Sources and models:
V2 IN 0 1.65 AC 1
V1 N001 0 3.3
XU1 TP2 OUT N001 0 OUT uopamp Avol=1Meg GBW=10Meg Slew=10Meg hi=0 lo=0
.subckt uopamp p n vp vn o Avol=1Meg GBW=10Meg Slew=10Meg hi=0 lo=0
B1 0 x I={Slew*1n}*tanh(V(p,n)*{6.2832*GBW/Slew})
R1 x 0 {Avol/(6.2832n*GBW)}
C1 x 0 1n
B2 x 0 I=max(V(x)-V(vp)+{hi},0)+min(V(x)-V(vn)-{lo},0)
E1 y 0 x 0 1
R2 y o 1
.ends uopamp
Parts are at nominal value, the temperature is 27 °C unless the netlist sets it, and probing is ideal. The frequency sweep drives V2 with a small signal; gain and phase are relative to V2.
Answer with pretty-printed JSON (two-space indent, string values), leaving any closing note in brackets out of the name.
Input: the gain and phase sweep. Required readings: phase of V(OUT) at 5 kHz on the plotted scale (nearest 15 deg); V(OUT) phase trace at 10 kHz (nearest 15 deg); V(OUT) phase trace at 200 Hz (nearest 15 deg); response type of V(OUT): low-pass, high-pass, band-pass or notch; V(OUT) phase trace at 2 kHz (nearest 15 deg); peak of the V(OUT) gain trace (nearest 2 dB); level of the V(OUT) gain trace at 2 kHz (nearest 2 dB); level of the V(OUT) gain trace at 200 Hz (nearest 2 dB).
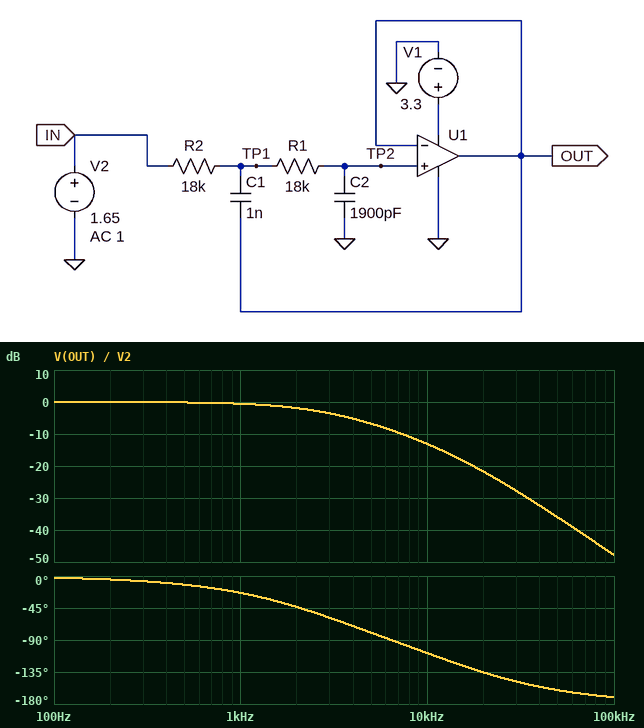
{
  "phase of V(OUT) at 5 kHz on the plotted scale": "-75 deg",
  "V(OUT) phase trace at 10 kHz": "-105 deg",
  "V(OUT) phase trace at 200 Hz": "0 deg",
  "response type of V(OUT): low-pass, high-pass, band-pass or notch": "low-pass",
  "V(OUT) phase trace at 2 kHz": "-45 deg",
  "peak of the V(OUT) gain trace": "0 dB",
  "level of the V(OUT) gain trace at 2 kHz": "-2 dB",
  "level of the V(OUT) gain trace at 200 Hz": "0 dB"
}
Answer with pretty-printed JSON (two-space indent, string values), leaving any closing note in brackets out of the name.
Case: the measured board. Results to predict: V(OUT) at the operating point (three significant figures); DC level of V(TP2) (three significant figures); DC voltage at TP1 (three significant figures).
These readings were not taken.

{
  "V(OUT) at the operating point": "1.65 V",
  "DC level of V(TP2)": "1.65 V",
  "DC voltage at TP1": "1.65 V"
}
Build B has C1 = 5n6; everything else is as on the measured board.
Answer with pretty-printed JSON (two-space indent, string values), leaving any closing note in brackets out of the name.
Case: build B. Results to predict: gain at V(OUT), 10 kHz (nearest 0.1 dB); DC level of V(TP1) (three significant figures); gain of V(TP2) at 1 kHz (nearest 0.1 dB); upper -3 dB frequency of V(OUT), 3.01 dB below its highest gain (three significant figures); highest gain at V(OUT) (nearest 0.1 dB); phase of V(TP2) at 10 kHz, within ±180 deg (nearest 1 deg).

{
  "gain at V(OUT), 10 kHz": "-22.5 dB",
  "DC level of V(TP1)": "1.65 V",
  "gain of V(TP2) at 1 kHz": "0.3 dB",
  "upper -3 dB frequency of V(OUT), 3.01 dB below its highest gain": "3.05 kHz",
  "highest gain at V(OUT)": "0.5 dB",
  "phase of V(TP2) at 10 kHz, within ±180 deg": "-161 deg"
}
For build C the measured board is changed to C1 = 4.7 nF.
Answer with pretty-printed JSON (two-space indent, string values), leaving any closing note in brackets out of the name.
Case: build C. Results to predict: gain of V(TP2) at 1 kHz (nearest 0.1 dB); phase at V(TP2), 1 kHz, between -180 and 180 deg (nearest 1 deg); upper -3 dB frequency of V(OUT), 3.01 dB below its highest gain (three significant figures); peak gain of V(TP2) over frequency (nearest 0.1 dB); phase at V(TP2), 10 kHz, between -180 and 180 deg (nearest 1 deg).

{
  "gain of V(TP2) at 1 kHz": "0.1 dB",
  "phase at V(TP2), 1 kHz, between -180 and 180 deg": "-26 deg",
  "upper -3 dB frequency of V(OUT), 3.01 dB below its highest gain": "3.20 kHz",
  "peak gain of V(TP2) over frequency": "0.2 dB",
  "phase at V(TP2), 10 kHz, between -180 and 180 deg": "-158 deg"
}
